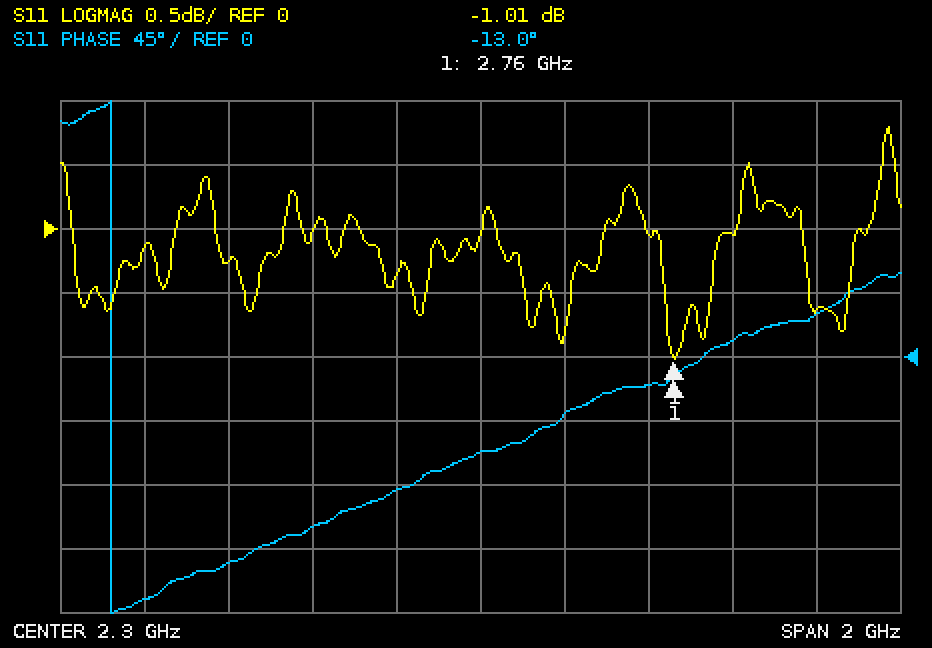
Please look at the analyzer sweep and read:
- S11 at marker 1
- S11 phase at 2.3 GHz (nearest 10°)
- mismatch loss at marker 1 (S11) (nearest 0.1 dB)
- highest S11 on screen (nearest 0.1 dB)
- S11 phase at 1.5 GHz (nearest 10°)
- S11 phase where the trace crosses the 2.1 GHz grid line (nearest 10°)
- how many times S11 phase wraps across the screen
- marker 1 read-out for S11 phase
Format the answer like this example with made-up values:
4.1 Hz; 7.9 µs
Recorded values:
-1.01 dB; -70°; 6.8 dB; 0.8 dB; -170°; -90°; 1; -13.0°
